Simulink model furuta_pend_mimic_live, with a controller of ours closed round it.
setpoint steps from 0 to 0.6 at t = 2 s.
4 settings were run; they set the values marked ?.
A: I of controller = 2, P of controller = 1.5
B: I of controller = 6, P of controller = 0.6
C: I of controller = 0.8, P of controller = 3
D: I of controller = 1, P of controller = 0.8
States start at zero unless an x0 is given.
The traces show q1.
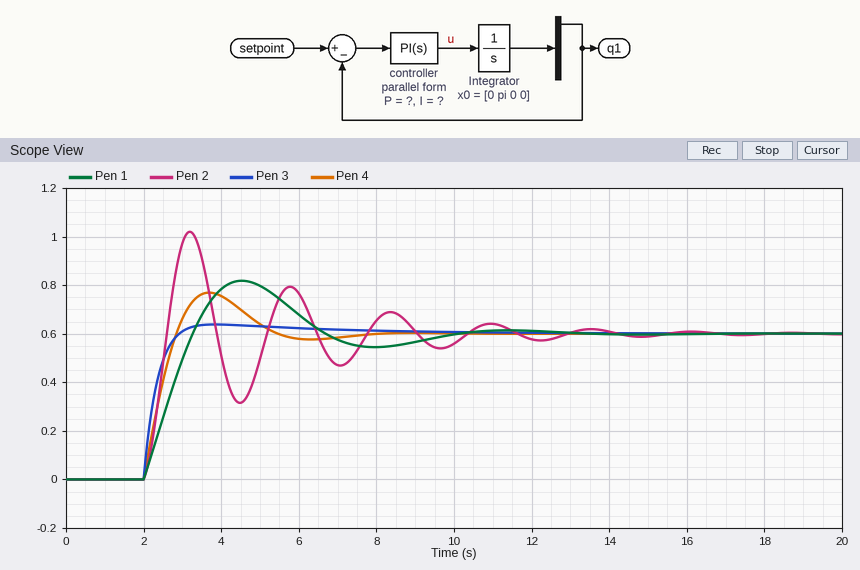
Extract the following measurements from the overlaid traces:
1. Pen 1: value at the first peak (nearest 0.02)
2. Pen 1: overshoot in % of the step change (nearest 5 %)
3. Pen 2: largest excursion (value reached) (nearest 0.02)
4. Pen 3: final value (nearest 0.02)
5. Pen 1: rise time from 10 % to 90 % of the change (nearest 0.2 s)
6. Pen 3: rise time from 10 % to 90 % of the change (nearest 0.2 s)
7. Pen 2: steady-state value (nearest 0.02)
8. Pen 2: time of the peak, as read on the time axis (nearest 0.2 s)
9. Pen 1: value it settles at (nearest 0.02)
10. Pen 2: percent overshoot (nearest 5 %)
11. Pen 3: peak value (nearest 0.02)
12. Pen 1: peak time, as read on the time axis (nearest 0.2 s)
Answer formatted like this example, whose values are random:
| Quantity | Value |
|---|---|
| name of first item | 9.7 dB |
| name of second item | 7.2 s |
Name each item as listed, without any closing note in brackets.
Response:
| Quantity | Value |
|---|---|
| Pen 1: value at the first peak | 0.82 |
| Pen 1: overshoot in % of the step change | 35 % |
| Pen 2: largest excursion (value reached) | 1.02 |
| Pen 3: final value | 0.60 |
| Pen 1: rise time from 10 % to 90 % of the change | 1.0 s |
| Pen 3: rise time from 10 % to 90 % of the change | 0.6 s |
| Pen 2: steady-state value | 0.60 |
| Pen 2: time of the peak, as read on the time axis | 3.2 s |
| Pen 1: value it settles at | 0.60 |
| Pen 2: percent overshoot | 70 % |
| Pen 3: peak value | 0.64 |
| Pen 1: peak time, as read on the time axis | 4.6 s |
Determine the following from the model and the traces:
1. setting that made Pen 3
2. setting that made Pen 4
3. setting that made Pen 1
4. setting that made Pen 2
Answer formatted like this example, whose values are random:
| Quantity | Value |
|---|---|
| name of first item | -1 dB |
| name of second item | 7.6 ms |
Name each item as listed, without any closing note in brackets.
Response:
| Quantity | Value |
|---|---|
| setting that made Pen 3 | C |
| setting that made Pen 4 | A |
| setting that made Pen 1 | D |
| setting that made Pen 2 | B |
